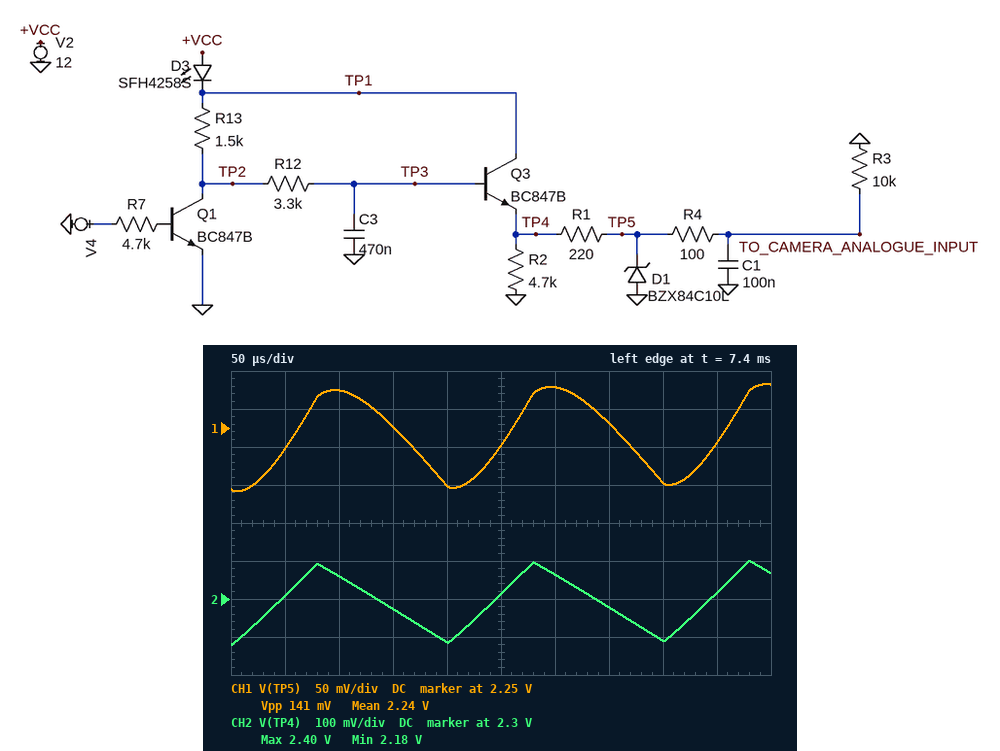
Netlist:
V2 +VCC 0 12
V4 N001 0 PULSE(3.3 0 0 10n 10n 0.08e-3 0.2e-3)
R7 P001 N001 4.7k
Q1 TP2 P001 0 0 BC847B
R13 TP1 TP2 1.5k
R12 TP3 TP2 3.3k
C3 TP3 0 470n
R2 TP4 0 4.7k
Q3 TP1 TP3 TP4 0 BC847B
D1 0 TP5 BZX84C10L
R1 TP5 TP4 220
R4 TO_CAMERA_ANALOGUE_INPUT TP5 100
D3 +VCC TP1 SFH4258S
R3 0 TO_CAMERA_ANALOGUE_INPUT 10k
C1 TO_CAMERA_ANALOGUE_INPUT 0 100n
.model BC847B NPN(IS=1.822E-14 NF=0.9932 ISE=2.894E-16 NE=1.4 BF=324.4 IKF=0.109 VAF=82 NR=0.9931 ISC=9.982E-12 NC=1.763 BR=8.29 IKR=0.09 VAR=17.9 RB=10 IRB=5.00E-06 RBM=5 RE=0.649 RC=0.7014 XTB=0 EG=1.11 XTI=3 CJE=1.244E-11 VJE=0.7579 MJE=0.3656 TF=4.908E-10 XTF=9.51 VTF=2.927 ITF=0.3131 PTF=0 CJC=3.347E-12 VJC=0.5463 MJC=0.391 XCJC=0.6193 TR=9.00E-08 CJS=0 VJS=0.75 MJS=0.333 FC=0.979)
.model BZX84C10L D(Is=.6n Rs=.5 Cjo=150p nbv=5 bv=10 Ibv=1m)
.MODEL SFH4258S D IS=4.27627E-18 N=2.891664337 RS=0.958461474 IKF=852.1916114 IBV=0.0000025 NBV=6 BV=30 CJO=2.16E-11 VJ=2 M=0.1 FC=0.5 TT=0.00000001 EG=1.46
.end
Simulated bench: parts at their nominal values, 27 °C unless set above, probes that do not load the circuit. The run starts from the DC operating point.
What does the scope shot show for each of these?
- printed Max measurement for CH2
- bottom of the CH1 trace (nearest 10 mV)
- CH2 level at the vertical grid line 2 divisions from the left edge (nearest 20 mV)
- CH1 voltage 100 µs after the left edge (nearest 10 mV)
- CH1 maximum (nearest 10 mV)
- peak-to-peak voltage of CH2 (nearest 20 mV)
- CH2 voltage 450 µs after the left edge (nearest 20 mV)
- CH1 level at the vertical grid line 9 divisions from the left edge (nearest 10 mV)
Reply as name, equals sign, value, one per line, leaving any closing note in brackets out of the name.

printed Max measurement for CH2 = 2.40 V
bottom of the CH1 trace = 2.17 V
CH2 level at the vertical grid line 2 divisions from the left edge = 2.36 V
CH1 voltage 100 µs after the left edge = 2.30 V
CH1 maximum = 2.31 V
peak-to-peak voltage of CH2 = 220 mV
CH2 voltage 450 µs after the left edge = 2.32 V
CH1 level at the vertical grid line 9 divisions from the left edge = 2.23 V
